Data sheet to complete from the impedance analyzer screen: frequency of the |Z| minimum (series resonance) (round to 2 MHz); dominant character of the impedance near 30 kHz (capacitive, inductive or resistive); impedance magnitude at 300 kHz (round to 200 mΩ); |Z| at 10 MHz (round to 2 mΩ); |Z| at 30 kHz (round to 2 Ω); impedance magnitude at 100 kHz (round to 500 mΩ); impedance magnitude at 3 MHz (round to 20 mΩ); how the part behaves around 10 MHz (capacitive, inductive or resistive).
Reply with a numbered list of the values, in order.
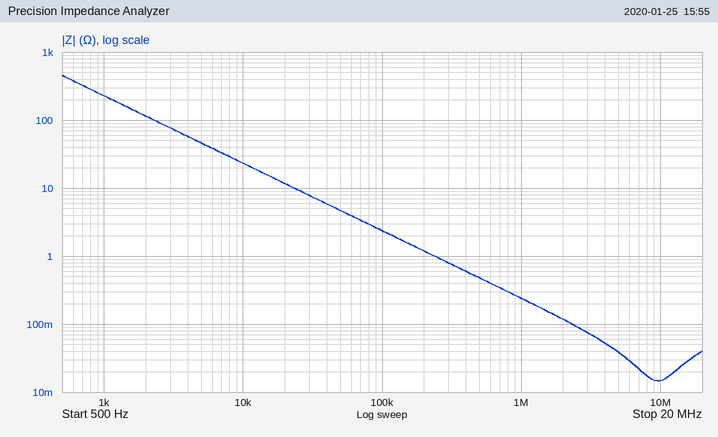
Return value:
1. 10 MHz
2. capacitive
3. 800 mΩ
4. 14 mΩ
5. 8 Ω
6. 2.5 Ω
7. 80 mΩ
8. resistive
